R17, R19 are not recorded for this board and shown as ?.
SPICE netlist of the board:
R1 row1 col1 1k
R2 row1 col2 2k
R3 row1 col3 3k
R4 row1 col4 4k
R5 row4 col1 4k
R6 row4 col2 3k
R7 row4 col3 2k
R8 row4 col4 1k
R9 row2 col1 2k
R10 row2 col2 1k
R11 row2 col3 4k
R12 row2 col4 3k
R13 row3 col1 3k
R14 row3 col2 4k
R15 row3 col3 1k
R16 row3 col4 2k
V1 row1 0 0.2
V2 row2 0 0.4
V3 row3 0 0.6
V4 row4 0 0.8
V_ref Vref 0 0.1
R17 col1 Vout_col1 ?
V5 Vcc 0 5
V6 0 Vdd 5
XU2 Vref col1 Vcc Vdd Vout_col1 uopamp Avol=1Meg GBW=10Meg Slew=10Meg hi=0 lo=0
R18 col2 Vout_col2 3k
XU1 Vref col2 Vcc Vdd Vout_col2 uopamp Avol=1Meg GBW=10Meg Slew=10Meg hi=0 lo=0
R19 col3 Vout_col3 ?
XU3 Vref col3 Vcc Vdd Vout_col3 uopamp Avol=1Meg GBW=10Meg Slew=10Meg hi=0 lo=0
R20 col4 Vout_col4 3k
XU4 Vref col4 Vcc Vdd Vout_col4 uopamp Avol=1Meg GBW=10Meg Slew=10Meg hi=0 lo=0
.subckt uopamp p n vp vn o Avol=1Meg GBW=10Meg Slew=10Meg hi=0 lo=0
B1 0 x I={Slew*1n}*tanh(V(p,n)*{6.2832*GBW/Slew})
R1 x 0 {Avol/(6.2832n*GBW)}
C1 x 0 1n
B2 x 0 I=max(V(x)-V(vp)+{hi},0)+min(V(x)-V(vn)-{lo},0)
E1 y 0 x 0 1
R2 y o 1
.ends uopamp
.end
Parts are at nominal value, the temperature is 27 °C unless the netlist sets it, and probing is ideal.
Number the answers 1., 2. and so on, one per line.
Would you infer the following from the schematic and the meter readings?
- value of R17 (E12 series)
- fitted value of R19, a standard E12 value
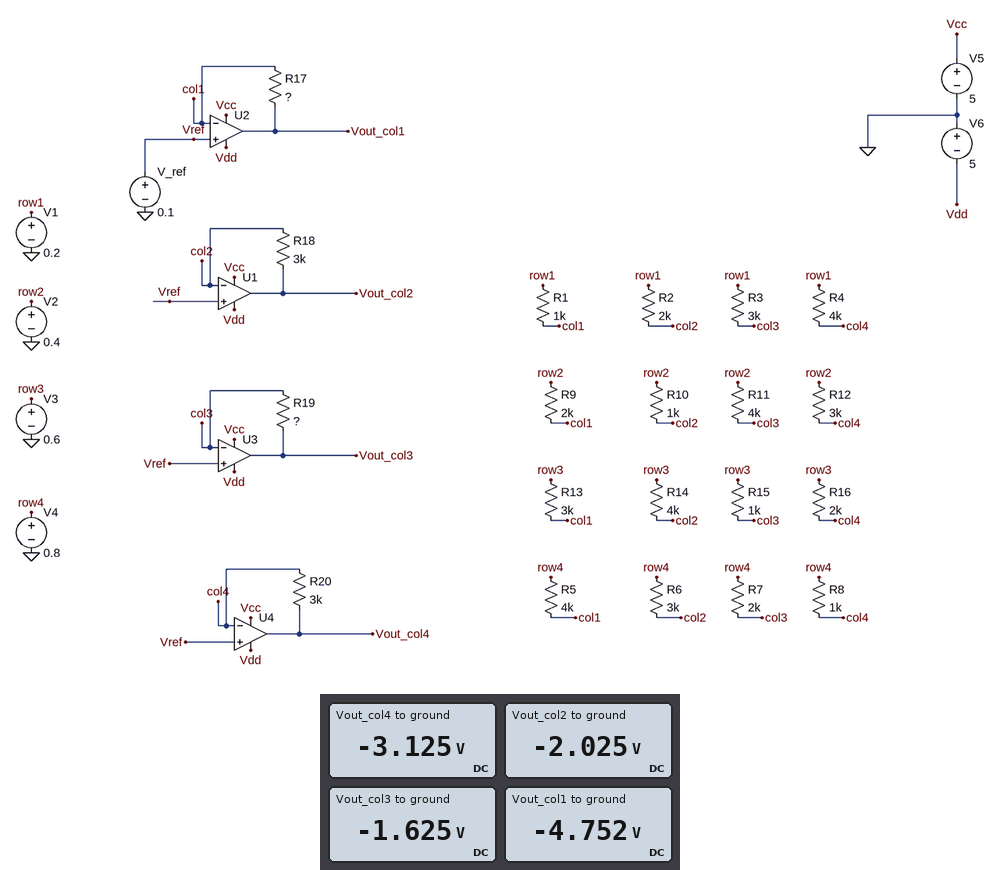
1. 8.2 kΩ
2. 1.8 kΩ
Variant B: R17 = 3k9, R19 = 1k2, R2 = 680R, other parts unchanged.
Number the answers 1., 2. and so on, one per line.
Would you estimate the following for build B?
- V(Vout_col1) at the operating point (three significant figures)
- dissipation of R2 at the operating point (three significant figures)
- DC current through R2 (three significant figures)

1. -2.21 V
2. 14.7 µW
3. 147 µA
